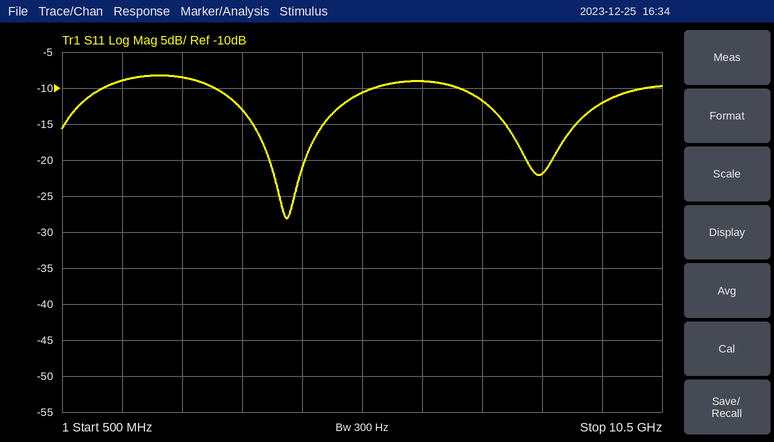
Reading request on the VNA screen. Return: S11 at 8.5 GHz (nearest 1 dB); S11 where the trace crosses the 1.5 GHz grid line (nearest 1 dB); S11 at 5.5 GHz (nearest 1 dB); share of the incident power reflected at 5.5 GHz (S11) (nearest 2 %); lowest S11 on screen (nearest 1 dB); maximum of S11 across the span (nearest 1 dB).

-22 dB
-9 dB
-11 dB
8 %
-28 dB
-8 dB
